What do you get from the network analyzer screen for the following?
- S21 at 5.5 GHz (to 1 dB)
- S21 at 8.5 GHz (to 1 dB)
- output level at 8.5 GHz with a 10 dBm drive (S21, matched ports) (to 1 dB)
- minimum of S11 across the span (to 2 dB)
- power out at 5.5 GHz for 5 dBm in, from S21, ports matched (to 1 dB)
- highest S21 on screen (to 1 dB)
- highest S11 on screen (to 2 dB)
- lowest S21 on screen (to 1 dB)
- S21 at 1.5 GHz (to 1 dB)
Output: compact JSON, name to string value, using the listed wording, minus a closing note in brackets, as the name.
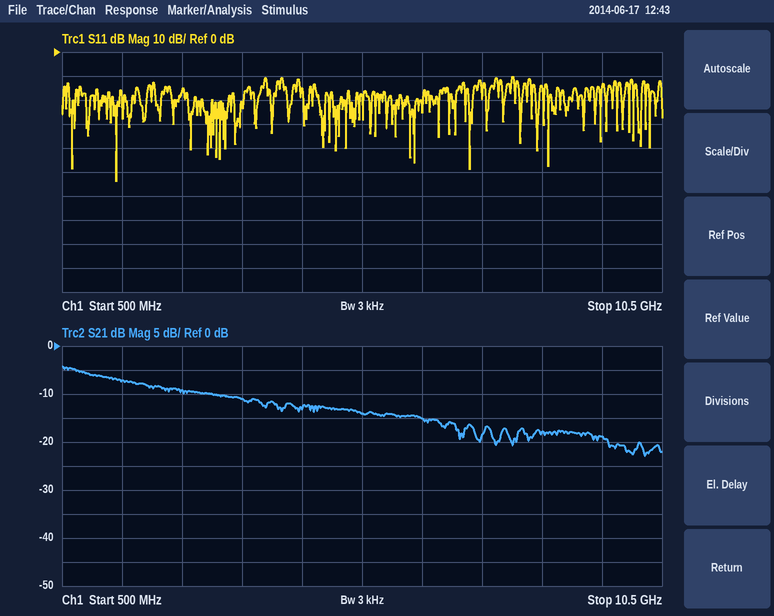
{"S21 at 5.5 GHz": "-14 dB", "S21 at 8.5 GHz": "-18 dB", "output level at 8.5 GHz with a 10 dBm drive (S21, matched ports)": "-8 dBm", "minimum of S11 across the span": "-54 dB", "power out at 5.5 GHz for 5 dBm in, from S21, ports matched": "-9 dBm", "highest S21 on screen": "-4 dB", "highest S11 on screen": "-10 dB", "lowest S21 on screen": "-23 dB", "S21 at 1.5 GHz": "-7 dB"}
